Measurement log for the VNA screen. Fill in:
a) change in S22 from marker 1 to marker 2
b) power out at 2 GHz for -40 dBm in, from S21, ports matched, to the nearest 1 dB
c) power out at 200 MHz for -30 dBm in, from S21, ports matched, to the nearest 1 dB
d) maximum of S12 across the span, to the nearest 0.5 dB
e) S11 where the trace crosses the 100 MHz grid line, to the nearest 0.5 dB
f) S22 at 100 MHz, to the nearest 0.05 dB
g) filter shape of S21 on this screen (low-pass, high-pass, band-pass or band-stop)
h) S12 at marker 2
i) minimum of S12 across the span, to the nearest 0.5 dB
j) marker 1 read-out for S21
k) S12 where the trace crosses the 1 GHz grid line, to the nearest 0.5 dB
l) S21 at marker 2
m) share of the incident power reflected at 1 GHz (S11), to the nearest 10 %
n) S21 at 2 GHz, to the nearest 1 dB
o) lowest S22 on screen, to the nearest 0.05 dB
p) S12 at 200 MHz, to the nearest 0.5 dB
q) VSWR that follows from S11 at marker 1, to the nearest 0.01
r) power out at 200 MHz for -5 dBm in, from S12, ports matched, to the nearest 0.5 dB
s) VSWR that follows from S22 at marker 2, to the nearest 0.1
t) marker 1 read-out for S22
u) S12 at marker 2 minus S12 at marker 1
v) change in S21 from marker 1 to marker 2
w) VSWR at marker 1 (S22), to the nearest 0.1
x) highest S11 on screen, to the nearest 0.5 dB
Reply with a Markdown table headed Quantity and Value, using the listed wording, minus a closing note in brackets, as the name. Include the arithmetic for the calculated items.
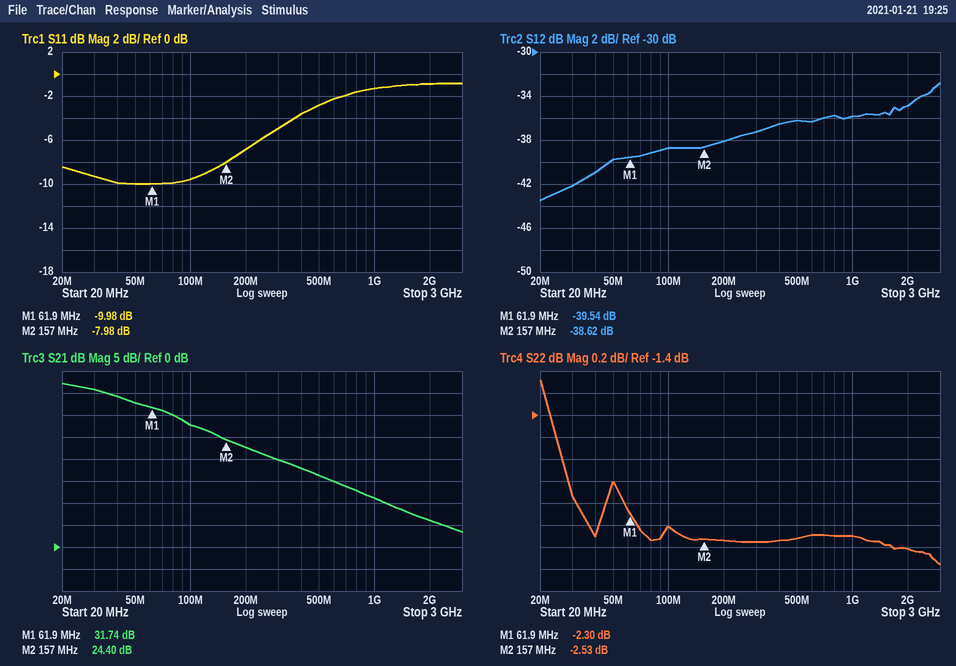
| Quantity | Value |
|---|---|
| change in S22 from marker 1 to marker 2 | -2.53 − (-2.3) = -0.23 dB |
| power out at 2 GHz for -40 dBm in, from S21, ports matched, to the nearest 1 dB | -40 dBm + (6 dB) = -34 dBm |
| power out at 200 MHz for -30 dBm in, from S21, ports matched, to the nearest 1 dB | -30 dBm + (23 dB) = -7 dBm |
| maximum of S12 across the span, to the nearest 0.5 dB | -33.0 dB |
| S11 where the trace crosses the 100 MHz grid line, to the nearest 0.5 dB | -9.5 dB |
| S22 at 100 MHz, to the nearest 0.05 dB | -2.40 dB |
| filter shape of S21 on this screen | low-pass |
| S12 at marker 2 | -38.62 dB |
| minimum of S12 across the span, to the nearest 0.5 dB | -43.5 dB |
| marker 1 read-out for S21 | 31.74 dB |
| S12 where the trace crosses the 1 GHz grid line, to the nearest 0.5 dB | -36.0 dB |
| S21 at marker 2 | 24.40 dB |
| share of the incident power reflected at 1 GHz (S11), to the nearest 10 % | 10^(-1.5/10) ≈ 70.8 %, so 70 % to the nearest 10 % |
| S21 at 2 GHz, to the nearest 1 dB | 6 dB |
| lowest S22 on screen, to the nearest 0.05 dB | -2.75 dB |
| S12 at 200 MHz, to the nearest 0.5 dB | -38.0 dB |
| VSWR that follows from S11 at marker 1, to the nearest 0.01 | (1 + 0.3170)/(1 − 0.3170) ≈ 1.93 |
| power out at 200 MHz for -5 dBm in, from S12, ports matched, to the nearest 0.5 dB | -5 dBm + (-38.0 dB) = -43.0 dBm |
| VSWR that follows from S22 at marker 2, to the nearest 0.1 | (1 + 0.7473)/(1 − 0.7473) ≈ 6.9 |
| marker 1 read-out for S22 | -2.30 dB |
| S12 at marker 2 minus S12 at marker 1 | -38.62 − (-39.54) = 0.92 dB |
| change in S21 from marker 1 to marker 2 | 24.4 − (31.74) = -7.34 dB |
| VSWR at marker 1 (S22), to the nearest 0.1 | (1 + 0.7674)/(1 − 0.7674) ≈ 7.6 |
| highest S11 on screen, to the nearest 0.5 dB | -1.0 dB |
